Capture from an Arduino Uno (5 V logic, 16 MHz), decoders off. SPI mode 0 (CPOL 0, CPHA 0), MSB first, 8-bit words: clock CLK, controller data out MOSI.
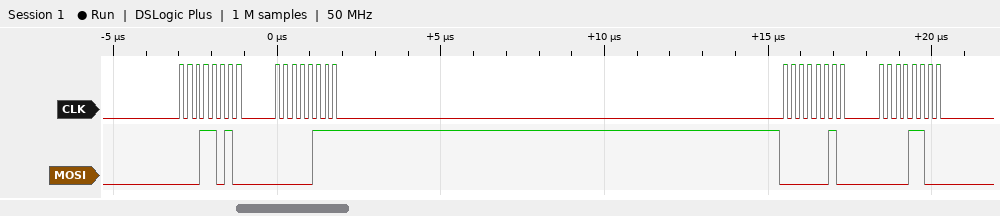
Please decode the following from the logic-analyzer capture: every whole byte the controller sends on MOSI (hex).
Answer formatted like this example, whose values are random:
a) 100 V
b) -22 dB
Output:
a) 0x1A 0x07 0x02 0x0C
